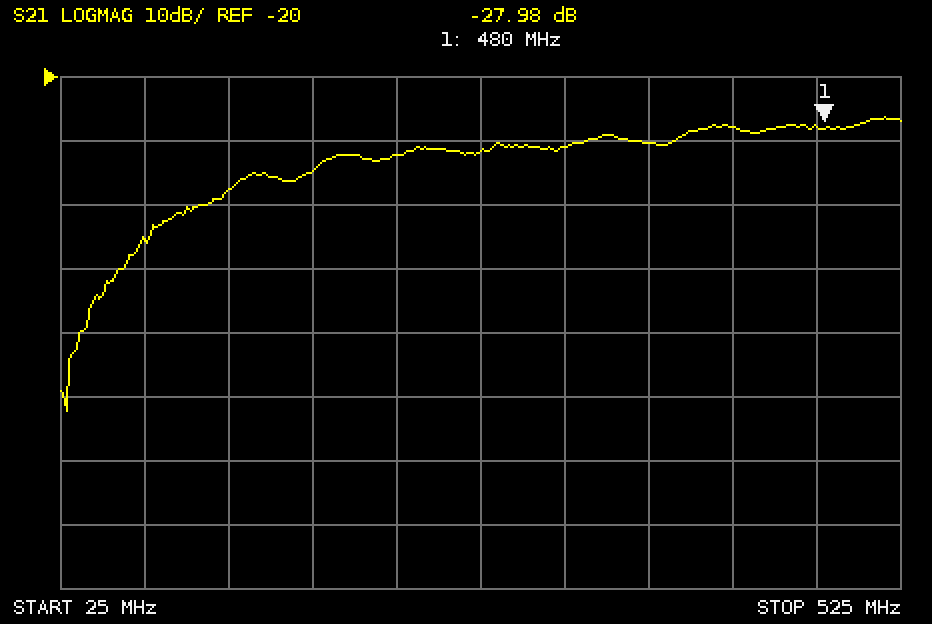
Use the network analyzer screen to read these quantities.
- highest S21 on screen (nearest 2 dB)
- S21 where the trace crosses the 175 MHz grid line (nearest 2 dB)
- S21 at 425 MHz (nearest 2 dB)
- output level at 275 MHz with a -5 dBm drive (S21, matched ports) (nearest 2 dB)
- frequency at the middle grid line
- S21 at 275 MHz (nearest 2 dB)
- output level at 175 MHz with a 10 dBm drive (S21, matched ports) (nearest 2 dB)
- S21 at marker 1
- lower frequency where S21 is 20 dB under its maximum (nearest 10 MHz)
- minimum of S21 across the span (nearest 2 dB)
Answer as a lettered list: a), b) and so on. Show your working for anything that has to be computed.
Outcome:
a) -26 dB
b) -34 dB
c) -28 dB
d) -5 dBm + (-32 dB) = -36 dBm
e) 275 MHz
f) -32 dB
g) 10 dBm + (-34 dB) = -24 dBm
h) -27.98 dB
i) 70 MHz
j) -72 dB
